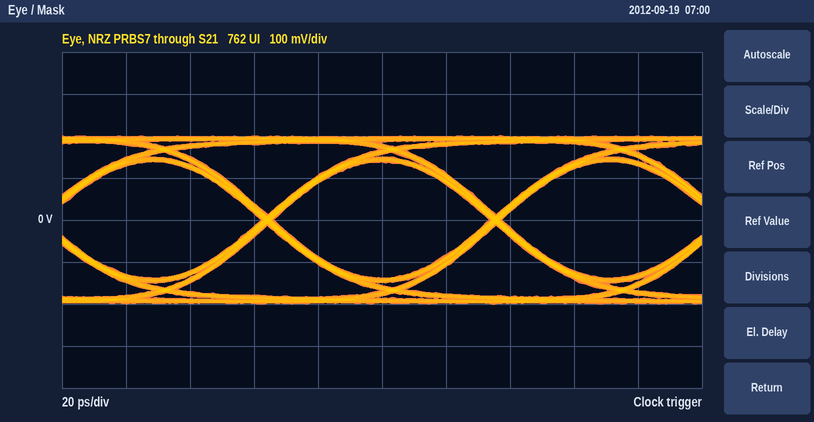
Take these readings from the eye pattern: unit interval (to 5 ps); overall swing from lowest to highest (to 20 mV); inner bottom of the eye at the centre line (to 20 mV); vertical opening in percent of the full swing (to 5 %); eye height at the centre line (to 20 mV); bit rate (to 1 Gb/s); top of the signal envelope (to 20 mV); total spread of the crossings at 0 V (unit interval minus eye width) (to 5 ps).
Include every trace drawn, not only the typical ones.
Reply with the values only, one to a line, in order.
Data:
70 ps
400 mV
-140 mV
70 %
280 mV
14 Gb/s
200 mV
5 ps
